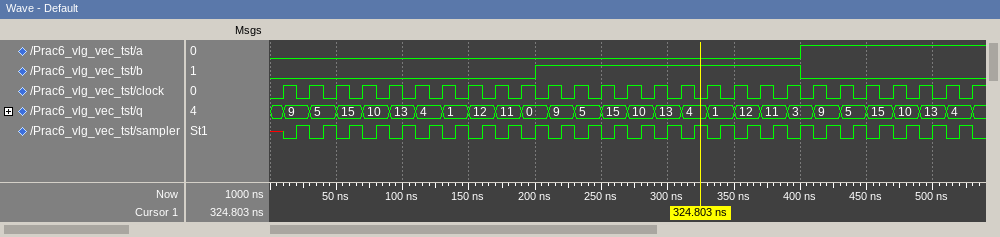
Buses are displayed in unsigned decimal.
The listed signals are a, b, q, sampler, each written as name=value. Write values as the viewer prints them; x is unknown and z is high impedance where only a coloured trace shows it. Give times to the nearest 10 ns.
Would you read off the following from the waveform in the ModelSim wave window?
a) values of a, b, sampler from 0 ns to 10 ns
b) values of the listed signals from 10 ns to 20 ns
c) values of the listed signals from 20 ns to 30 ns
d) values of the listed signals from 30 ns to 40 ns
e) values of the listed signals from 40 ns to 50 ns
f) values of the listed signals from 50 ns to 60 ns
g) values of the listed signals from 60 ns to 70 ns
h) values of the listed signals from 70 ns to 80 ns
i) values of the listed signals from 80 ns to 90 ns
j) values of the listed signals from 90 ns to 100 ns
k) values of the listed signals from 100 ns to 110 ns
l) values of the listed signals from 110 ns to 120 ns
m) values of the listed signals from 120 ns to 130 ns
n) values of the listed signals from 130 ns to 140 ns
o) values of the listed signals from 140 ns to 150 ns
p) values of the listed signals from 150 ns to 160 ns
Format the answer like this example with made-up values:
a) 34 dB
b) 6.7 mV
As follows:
a) a=0, b=0, sampler=x
b) a=0, b=0, q=9, sampler=0
c) a=0, b=0, q=9, sampler=1
d) a=0, b=0, q=5, sampler=0
e) a=0, b=0, q=5, sampler=1
f) a=0, b=0, q=15, sampler=0
g) a=0, b=0, q=15, sampler=1
h) a=0, b=0, q=10, sampler=0
i) a=0, b=0, q=10, sampler=1
j) a=0, b=0, q=13, sampler=0
k) a=0, b=0, q=13, sampler=1
l) a=0, b=0, q=4, sampler=0
m) a=0, b=0, q=4, sampler=1
n) a=0, b=0, q=1, sampler=0
o) a=0, b=0, q=1, sampler=1
p) a=0, b=0, q=12, sampler=0
